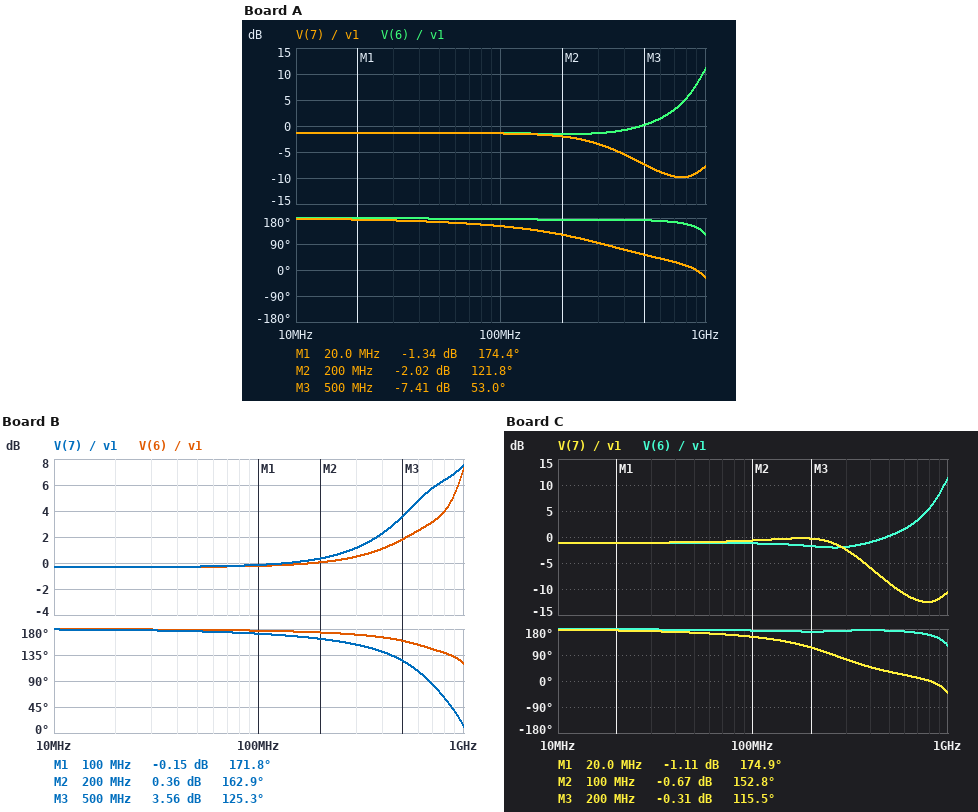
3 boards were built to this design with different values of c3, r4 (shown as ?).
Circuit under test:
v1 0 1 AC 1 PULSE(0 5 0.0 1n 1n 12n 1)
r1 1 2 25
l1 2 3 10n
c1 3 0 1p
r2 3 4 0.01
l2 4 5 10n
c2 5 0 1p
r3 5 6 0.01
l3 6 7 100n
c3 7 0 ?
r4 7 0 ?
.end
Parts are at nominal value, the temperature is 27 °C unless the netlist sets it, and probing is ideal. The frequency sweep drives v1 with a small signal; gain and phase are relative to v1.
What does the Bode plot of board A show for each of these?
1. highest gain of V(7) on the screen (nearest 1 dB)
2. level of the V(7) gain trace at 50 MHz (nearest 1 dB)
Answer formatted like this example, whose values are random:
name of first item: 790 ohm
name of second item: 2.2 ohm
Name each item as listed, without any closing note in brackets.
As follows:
highest gain of V(7) on the screen: -1 dB
level of the V(7) gain trace at 50 MHz: -1 dB
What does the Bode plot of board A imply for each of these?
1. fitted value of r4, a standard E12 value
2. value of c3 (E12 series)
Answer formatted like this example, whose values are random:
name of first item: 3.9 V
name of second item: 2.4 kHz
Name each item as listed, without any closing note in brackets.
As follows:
fitted value of r4, a standard E12 value: 150 Ω
value of c3: 2.2 pF
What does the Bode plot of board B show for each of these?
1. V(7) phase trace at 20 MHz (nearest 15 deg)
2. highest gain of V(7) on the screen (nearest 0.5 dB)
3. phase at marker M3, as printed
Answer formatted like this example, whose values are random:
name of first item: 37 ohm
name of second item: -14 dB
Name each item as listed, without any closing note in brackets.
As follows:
V(7) phase trace at 20 MHz: 180 deg
highest gain of V(7) on the screen: 7.5 dB
phase at marker M3, as printed: 125.3 deg
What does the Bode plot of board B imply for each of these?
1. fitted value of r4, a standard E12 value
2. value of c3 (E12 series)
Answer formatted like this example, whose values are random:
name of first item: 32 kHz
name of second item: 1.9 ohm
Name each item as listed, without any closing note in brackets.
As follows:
fitted value of r4, a standard E12 value: 680 Ω
value of c3: 330 fF
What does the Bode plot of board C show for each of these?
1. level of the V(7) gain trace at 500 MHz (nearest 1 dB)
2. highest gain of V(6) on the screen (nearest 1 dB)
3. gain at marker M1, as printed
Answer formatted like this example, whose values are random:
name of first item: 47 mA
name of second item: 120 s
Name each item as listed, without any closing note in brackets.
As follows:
level of the V(7) gain trace at 500 MHz: -9 dB
highest gain of V(6) on the screen: 11 dB
gain at marker M1, as printed: -1.11 dB
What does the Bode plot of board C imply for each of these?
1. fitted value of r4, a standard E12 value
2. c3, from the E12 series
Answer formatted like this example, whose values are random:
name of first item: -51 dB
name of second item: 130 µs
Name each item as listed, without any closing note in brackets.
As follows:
fitted value of r4, a standard E12 value: 180 Ω
c3, from the E12 series: 3.3 pF
